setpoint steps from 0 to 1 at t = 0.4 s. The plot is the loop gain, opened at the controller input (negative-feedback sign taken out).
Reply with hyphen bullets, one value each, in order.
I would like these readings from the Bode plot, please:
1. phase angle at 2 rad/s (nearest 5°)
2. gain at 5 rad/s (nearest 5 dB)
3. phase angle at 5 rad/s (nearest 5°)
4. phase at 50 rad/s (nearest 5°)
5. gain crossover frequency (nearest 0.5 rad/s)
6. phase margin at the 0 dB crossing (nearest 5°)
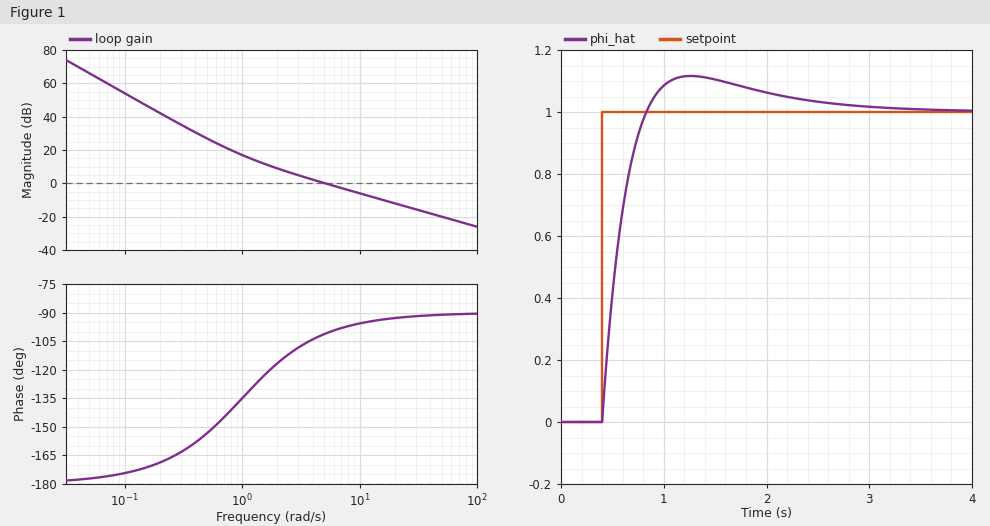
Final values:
- -115°
- 0 dB
- -100°
- -90°
- 5.0 rad/s
- 80°
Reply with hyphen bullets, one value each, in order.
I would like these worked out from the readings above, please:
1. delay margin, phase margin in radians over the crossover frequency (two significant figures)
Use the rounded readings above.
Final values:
- 0.28 s
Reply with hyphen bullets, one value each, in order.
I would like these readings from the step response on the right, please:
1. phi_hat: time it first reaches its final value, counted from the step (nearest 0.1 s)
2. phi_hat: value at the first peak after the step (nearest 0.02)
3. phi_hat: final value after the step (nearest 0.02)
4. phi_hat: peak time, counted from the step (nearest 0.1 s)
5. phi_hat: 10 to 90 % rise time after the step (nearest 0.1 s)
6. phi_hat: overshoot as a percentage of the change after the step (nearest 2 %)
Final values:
- 0.4 s
- 1.12
- 1.00
- 0.9 s
- 0.3 s
- 12 %
